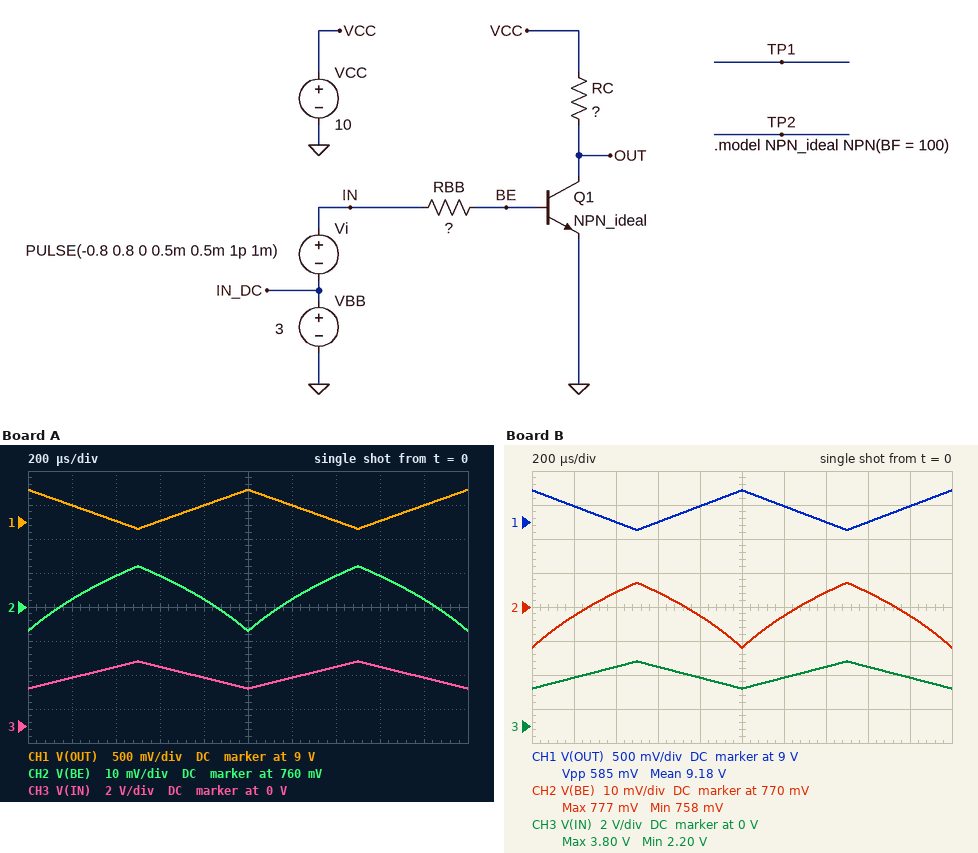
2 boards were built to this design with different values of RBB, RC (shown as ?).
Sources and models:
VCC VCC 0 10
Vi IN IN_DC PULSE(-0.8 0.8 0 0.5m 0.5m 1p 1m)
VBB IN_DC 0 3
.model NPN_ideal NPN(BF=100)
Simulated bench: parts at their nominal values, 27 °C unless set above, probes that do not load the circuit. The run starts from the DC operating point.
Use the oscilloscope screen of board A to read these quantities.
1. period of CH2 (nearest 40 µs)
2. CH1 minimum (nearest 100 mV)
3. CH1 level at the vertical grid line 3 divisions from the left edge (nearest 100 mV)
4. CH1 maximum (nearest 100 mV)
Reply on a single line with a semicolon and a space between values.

1.00 ms; 8.9 V; 9.0 V; 9.5 V
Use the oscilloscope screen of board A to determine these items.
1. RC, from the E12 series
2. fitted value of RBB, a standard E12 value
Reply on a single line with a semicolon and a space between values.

1.2 kΩ; 330 kΩ
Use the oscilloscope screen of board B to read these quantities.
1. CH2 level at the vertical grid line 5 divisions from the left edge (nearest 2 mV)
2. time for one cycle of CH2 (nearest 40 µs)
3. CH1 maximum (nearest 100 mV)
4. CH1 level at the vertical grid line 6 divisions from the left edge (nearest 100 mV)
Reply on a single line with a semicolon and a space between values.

758 mV; 1.00 ms; 9.5 V; 9.2 V
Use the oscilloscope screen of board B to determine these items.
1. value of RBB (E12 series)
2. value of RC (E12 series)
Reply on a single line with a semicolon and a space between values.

270 kΩ; 1 kΩ
